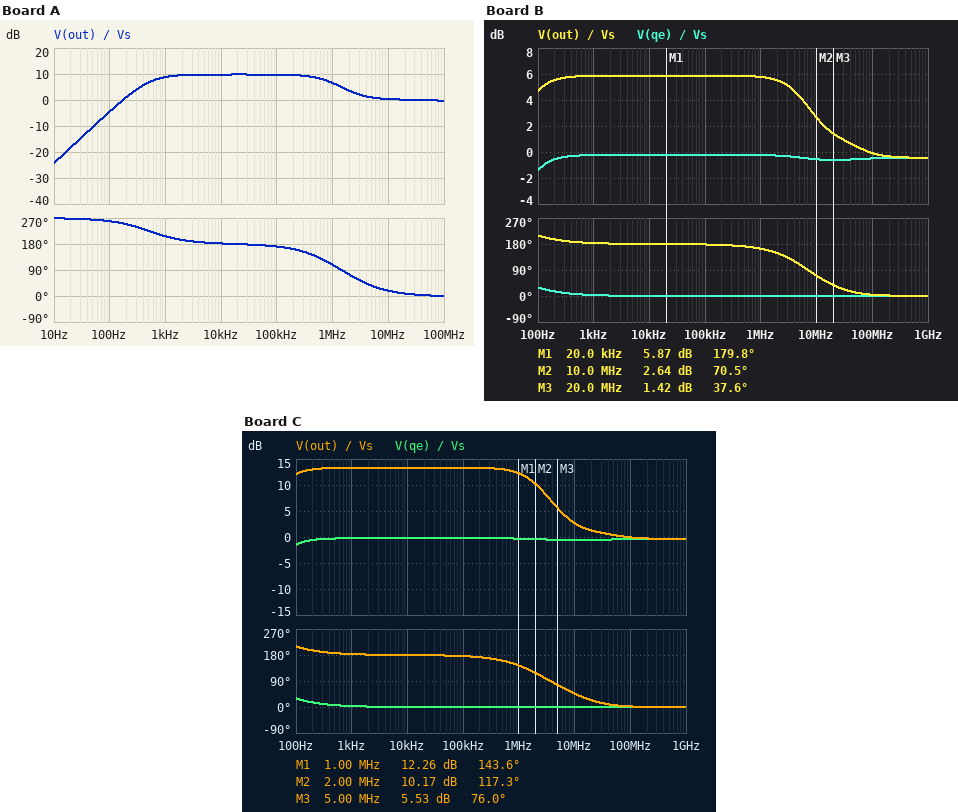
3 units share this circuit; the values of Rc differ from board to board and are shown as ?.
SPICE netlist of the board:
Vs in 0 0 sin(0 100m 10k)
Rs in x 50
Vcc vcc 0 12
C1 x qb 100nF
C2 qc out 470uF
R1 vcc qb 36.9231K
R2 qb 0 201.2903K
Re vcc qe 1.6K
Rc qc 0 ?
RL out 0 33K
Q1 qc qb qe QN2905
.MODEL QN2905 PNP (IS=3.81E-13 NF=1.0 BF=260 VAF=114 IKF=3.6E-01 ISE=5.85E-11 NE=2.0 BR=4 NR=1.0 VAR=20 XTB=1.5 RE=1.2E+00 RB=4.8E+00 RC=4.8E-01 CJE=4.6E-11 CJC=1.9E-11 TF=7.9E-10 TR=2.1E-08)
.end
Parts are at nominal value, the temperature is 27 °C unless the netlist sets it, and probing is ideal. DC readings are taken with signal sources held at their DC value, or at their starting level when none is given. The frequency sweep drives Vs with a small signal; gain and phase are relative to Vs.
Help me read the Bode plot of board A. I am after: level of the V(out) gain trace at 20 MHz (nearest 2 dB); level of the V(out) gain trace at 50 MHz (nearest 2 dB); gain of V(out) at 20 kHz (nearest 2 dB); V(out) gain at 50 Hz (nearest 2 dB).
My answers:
0 dB
0 dB
10 dB
-10 dB
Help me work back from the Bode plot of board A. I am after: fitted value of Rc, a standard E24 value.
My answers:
16 kΩ
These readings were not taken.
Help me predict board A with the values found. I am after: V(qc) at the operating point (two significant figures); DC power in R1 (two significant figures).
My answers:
11 V
73 µW
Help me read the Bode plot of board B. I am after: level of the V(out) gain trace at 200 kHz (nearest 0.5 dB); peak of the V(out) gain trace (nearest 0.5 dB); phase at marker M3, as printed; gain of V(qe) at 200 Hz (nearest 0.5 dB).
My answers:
6.0 dB
6.0 dB
37.6 deg
-0.5 dB
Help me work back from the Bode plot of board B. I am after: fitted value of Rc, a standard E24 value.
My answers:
3.6 kΩ
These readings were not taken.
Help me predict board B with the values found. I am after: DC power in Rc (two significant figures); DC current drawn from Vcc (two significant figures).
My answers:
1.8 mW
760 µA
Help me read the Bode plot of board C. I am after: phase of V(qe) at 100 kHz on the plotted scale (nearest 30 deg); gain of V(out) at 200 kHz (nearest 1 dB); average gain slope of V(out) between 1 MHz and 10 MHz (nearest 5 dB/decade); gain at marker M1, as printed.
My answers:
0 deg
13 dB
-10 dB/decade
12.26 dB
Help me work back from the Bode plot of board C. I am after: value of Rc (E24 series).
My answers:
10 kΩ
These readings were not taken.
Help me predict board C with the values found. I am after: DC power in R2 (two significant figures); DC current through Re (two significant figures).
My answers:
530 µW
710 µA
